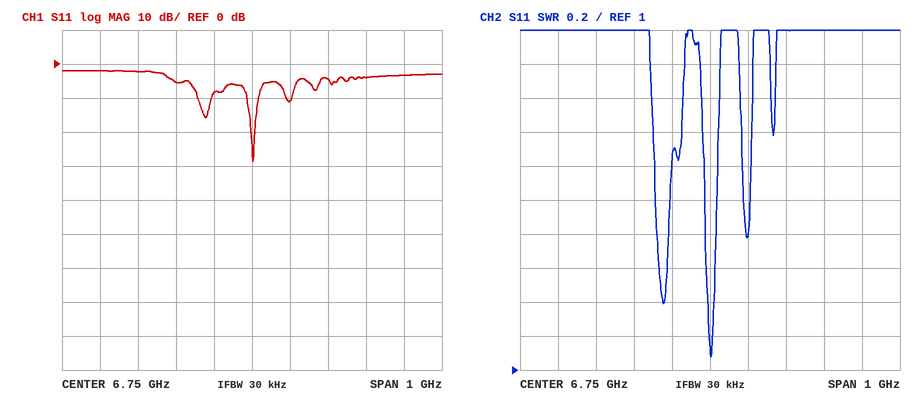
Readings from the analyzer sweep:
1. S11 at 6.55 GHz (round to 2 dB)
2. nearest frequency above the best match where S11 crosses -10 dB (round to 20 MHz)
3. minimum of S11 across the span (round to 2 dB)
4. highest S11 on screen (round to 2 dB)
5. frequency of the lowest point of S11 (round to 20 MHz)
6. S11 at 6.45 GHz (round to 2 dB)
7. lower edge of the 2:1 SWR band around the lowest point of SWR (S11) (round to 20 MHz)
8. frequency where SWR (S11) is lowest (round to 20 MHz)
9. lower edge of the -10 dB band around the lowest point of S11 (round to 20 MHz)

-6 dB
6.76 GHz
-28 dB
-2 dB
6.76 GHz
-2 dB
6.74 GHz
6.76 GHz
6.74 GHz
